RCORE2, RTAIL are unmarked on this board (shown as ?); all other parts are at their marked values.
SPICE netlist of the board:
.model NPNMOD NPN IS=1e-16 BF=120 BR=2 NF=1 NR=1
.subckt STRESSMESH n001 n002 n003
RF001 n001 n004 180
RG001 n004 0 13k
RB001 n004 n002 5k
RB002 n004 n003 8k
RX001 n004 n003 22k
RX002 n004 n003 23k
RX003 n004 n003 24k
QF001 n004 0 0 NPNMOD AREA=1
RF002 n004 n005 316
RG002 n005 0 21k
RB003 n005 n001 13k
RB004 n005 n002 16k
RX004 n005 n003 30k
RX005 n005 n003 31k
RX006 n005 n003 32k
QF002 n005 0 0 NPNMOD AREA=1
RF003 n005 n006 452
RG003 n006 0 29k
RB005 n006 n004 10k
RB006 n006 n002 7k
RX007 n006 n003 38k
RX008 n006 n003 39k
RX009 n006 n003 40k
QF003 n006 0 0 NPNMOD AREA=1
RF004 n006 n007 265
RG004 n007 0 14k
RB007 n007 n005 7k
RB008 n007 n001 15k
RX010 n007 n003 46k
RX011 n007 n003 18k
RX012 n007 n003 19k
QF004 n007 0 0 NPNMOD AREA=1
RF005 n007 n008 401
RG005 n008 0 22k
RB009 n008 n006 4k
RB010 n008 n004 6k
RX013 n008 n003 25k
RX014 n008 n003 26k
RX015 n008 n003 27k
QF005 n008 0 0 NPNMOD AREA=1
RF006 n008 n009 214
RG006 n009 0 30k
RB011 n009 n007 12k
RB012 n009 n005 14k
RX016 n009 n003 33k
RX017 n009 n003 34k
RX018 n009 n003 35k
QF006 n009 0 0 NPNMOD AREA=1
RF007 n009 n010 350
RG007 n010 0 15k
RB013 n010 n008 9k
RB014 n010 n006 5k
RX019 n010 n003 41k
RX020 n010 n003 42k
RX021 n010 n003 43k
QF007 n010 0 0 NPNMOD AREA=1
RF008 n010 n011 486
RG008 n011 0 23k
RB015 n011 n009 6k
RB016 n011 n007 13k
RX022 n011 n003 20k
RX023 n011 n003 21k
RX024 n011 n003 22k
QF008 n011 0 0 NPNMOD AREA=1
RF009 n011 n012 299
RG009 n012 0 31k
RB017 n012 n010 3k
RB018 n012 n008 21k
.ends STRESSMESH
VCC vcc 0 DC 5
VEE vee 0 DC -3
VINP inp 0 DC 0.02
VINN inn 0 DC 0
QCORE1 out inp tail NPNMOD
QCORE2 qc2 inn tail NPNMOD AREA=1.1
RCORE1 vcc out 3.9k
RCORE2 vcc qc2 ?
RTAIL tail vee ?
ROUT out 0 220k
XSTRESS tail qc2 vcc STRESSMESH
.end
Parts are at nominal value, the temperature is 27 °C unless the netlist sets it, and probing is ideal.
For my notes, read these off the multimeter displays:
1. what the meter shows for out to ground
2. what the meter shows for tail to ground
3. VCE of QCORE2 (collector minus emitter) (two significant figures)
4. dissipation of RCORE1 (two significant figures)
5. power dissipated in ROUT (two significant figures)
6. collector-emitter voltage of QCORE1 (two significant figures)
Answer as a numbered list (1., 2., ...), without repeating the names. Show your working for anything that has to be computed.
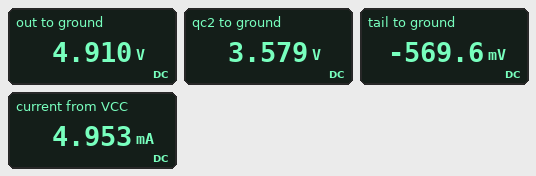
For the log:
1. 4.910 V
2. -569.6 mV
3. 3.579 V - (-569.6 mV) = 4.1 V
4. (5 V - 4.91 V)^2 / 3.9 kΩ = 2.1 µW
5. (4.91 V)^2 / 220 kΩ = 110 µW
6. 4.91 V - (-569.6 mV) = 5.5 V
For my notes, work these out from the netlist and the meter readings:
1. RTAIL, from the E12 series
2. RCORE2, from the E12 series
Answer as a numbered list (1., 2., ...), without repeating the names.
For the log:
1. 560 Ω
2. 1.2 kΩ
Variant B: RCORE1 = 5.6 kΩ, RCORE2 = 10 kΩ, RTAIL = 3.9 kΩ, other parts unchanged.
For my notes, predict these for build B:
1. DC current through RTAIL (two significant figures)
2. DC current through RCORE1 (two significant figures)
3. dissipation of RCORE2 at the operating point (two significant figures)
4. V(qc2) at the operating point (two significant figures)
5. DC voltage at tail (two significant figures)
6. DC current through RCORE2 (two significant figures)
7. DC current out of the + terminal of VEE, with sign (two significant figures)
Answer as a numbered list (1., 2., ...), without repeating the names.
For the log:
1. 1.3 mA
2. 22 µA
3. 410 µW
4. 3.0 V
5. 2.1 V
6. 200 µA
7. -1.3 mA
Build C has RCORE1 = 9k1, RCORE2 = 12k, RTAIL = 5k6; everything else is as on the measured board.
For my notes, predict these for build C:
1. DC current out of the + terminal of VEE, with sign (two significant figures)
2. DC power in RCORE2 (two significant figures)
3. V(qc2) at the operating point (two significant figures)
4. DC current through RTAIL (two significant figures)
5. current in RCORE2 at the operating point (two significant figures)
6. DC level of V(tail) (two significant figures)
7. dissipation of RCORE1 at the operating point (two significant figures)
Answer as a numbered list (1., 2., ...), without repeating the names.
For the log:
1. -980 µA
2. 290 µW
3. 3.1 V
4. 980 µA
5. 160 µA
6. 2.5 V
7. 4.3 µW
